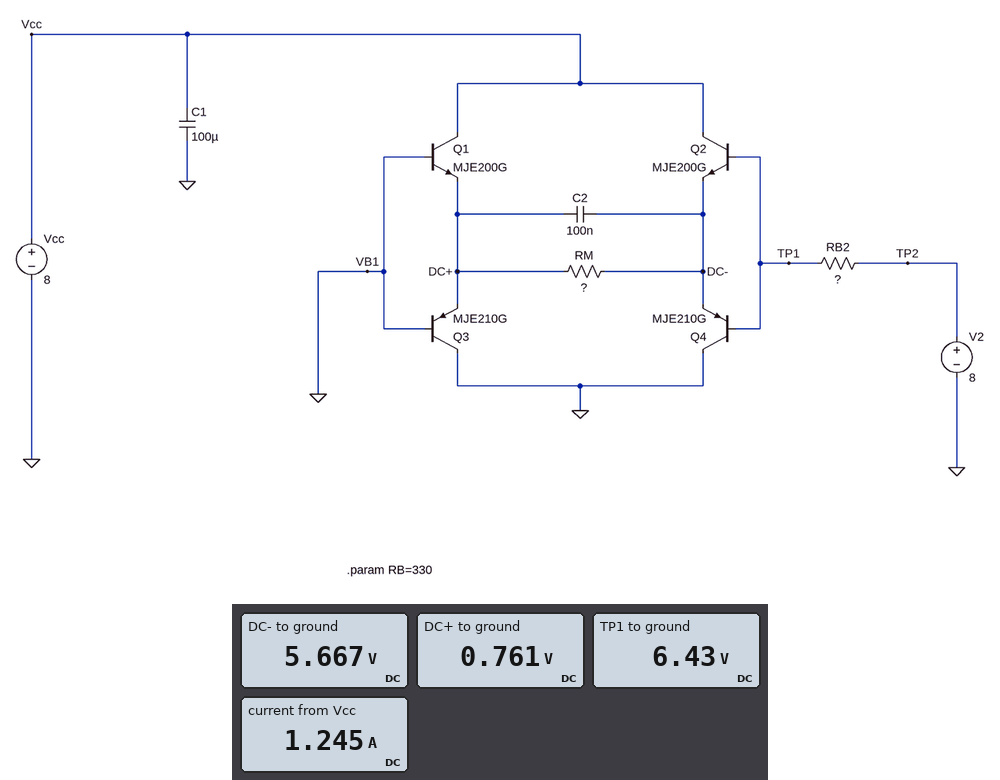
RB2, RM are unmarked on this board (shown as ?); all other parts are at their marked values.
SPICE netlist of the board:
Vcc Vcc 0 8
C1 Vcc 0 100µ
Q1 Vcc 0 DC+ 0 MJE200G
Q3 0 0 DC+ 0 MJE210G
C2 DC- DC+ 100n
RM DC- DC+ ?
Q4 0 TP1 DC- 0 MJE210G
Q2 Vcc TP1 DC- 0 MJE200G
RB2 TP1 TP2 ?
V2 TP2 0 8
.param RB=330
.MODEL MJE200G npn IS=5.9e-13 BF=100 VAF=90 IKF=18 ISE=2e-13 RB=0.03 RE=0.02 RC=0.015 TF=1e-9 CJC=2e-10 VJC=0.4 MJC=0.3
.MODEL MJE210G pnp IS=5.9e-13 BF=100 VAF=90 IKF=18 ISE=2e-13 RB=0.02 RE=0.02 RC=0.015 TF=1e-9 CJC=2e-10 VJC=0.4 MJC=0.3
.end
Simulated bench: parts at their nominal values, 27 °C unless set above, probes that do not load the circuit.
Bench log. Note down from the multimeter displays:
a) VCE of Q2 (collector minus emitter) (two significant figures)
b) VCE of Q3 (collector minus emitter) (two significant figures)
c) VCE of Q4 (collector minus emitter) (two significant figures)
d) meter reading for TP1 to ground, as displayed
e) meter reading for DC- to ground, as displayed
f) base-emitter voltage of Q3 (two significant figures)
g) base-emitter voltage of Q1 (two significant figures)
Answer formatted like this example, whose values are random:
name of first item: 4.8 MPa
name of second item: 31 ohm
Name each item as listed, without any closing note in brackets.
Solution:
VCE of Q2 (collector minus emitter): 2.3 V
VCE of Q3 (collector minus emitter): -760 mV
VCE of Q4 (collector minus emitter): -5.7 V
meter reading for TP1 to ground, as displayed: 6.43 V
meter reading for DC- to ground, as displayed: 5.667 V
base-emitter voltage of Q3: -760 mV
base-emitter voltage of Q1: -760 mV
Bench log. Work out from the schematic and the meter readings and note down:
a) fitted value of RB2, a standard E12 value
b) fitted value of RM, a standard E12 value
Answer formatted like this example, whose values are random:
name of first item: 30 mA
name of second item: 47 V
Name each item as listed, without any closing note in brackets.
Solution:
fitted value of RB2, a standard E12 value: 120 Ω
fitted value of RM, a standard E12 value: 3.9 Ω
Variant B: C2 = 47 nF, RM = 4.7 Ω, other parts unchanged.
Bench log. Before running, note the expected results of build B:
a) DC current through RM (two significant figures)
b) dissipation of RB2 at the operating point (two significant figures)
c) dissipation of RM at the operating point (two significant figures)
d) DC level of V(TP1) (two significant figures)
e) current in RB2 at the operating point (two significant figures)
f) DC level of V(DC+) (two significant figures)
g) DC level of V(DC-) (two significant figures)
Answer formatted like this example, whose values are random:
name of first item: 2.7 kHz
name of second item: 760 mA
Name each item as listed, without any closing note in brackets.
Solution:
DC current through RM: 1.1 A
dissipation of RB2 at the operating point: 15 mW
dissipation of RM at the operating point: 5.6 W
DC level of V(TP1): 6.6 V
current in RB2 at the operating point: 11 mA
DC level of V(DC+): 750 mV
DC level of V(DC-): 5.9 V
